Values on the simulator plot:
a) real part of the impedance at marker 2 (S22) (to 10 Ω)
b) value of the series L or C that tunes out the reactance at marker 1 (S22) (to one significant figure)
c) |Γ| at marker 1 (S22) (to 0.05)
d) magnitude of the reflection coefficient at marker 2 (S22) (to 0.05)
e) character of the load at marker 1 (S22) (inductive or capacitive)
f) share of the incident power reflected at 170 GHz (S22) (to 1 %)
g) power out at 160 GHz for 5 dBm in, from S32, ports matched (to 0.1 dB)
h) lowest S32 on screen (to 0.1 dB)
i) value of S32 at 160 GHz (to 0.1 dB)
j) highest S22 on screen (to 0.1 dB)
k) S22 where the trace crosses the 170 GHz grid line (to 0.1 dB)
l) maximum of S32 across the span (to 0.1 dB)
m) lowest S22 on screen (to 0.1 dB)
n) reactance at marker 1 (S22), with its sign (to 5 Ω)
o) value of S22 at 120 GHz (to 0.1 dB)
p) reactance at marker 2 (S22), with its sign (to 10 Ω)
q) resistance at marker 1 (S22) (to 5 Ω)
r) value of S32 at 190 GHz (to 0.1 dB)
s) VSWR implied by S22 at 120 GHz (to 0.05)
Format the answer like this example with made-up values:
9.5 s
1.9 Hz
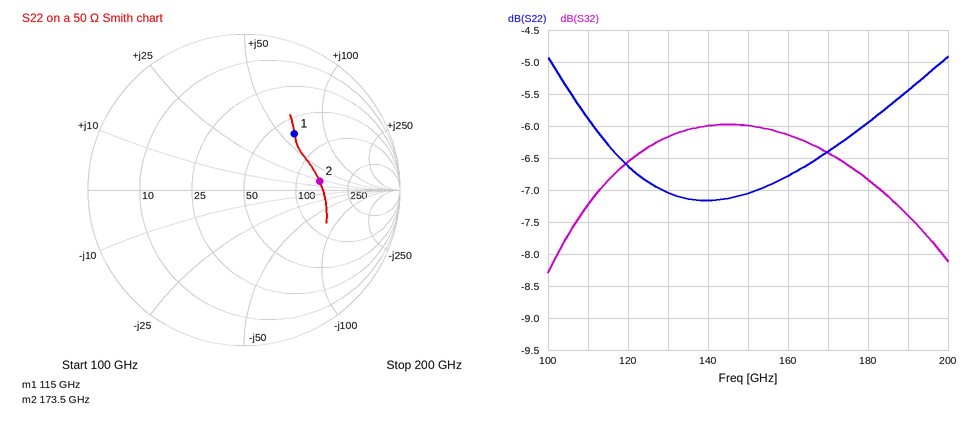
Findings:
140 Ω
20 fF
0.50
0.50
inductive
23 %
-1.1 dBm
-8.3 dB
-6.1 dB
-4.9 dB
-6.4 dB
-6.0 dB
-7.2 dB
+60 Ω
-6.6 dB
+20 Ω
65 Ω
-7.4 dB
2.75
